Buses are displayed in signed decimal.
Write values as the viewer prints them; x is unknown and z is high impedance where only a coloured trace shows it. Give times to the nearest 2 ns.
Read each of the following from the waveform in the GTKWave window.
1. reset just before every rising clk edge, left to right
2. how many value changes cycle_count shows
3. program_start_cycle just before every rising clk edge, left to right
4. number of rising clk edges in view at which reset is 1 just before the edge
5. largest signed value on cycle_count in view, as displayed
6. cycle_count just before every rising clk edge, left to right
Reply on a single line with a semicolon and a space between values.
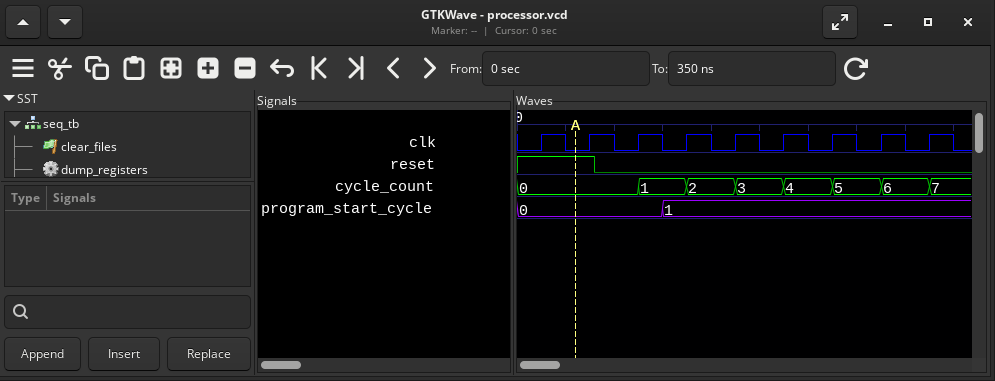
1 1 0 0 0 0 0 0 0; 7; 0, 0, 0, 1, 1, 1, 1, 1, 1; 2; 7; 0, 0, 0, 1, 2, 3, 4, 5, 6
